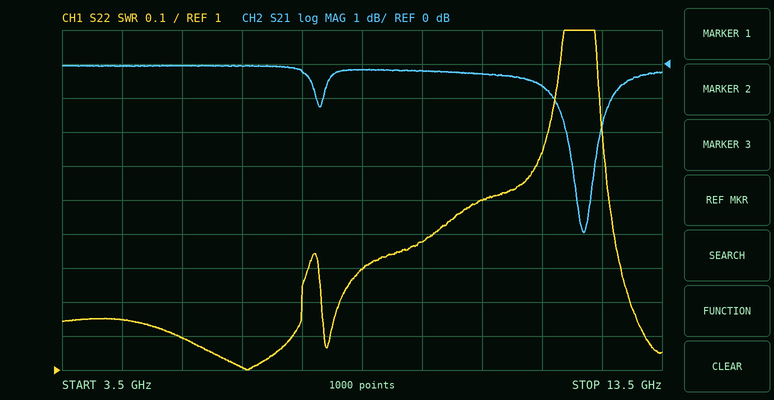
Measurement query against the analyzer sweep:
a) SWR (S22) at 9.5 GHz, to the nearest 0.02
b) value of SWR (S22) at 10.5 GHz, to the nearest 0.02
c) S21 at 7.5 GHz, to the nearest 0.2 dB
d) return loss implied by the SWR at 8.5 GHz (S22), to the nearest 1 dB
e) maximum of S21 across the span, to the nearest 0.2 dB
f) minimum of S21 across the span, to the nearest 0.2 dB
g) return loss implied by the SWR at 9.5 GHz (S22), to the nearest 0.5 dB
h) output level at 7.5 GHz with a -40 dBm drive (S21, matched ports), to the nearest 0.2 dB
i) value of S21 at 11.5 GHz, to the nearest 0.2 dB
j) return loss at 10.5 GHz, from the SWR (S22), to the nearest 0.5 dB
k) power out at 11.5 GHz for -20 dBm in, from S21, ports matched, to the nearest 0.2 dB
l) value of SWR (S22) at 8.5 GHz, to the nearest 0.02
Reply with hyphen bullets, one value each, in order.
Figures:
- 1.38
- 1.50
- -0.2 dB
- 18 dB
- 0.0 dB
- -5.0 dB
- 16.0 dB
- -40.2 dBm
- -0.6 dB
- 14.0 dB
- -20.6 dBm
- 1.30
